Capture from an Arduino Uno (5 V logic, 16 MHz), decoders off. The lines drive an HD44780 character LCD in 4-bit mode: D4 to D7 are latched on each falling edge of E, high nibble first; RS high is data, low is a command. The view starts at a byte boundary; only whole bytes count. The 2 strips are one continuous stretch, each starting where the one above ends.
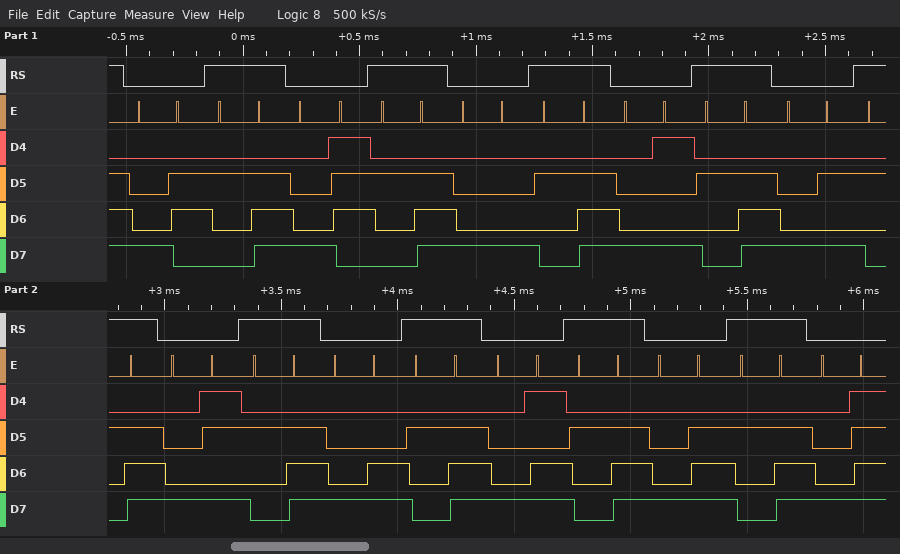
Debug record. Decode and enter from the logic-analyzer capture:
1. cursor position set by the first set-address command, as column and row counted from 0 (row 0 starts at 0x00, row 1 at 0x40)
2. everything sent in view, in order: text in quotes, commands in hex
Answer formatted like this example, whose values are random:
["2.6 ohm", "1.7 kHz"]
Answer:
["column 6, row 0", "0x86 \".\" 0x87 \".\" 0x88 \".\" 0x89 \".\" 0x8A \".\" 0x8B \".\" 0x8C \".\" 0x8D \".\" 0x8E \".\" 0x8F"]
